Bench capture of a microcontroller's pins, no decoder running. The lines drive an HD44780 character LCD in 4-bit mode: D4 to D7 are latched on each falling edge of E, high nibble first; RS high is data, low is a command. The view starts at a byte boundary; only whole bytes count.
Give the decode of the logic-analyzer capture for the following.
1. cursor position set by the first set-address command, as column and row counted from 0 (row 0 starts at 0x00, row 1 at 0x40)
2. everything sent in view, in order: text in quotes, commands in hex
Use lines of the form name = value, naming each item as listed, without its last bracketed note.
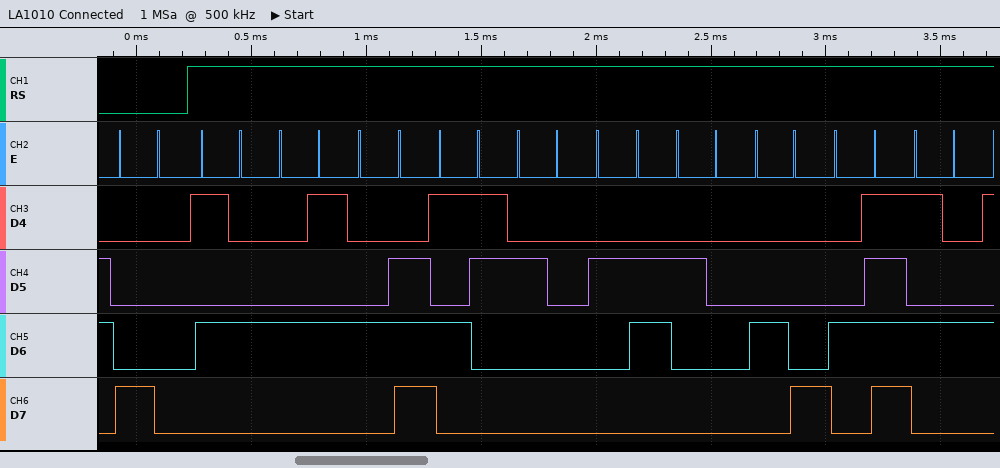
cursor position set by the first set-address command, as column and row counted from 0 = column 0, row 0
everything sent in view, in order: text in quotes, commands in hex = 0x80 "TENS & HOT"
